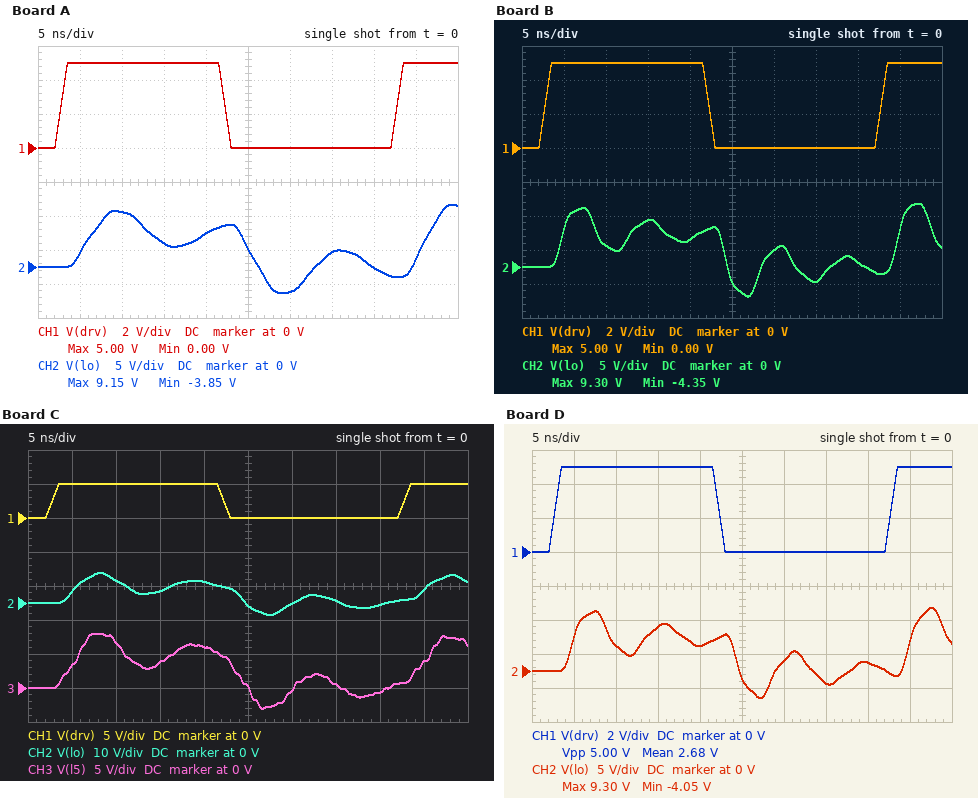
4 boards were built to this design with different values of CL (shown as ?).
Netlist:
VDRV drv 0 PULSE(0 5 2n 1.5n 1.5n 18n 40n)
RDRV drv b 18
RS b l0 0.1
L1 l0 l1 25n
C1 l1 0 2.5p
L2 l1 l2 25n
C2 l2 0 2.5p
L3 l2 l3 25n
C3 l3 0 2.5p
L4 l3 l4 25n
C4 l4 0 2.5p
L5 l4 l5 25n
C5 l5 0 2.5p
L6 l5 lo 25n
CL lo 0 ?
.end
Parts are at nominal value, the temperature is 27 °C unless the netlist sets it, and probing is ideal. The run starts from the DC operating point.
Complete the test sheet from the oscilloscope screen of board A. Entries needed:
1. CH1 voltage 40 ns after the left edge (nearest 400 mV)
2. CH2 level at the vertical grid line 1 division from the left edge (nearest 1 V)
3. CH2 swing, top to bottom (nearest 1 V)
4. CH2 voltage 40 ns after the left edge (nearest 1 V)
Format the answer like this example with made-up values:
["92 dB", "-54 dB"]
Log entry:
["0 V", "2 V", "13 V", "0 V"]
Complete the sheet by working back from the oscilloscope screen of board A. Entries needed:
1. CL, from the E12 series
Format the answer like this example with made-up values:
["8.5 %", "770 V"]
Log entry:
["27 pF"]
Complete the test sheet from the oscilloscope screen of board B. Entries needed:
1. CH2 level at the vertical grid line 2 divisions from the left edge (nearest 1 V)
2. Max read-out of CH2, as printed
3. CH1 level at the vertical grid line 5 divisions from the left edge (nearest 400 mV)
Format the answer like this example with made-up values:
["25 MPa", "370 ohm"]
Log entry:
["3 V", "9.30 V", "0 V"]
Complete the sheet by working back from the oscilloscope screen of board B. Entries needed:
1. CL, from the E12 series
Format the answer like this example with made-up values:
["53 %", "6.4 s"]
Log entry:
["6.8 pF"]
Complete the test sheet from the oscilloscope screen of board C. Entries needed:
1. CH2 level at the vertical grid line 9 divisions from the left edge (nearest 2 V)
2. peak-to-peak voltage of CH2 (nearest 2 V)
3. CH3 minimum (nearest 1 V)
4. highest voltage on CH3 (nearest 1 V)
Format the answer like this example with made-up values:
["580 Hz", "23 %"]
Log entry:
["4 V", "12 V", "-3 V", "8 V"]
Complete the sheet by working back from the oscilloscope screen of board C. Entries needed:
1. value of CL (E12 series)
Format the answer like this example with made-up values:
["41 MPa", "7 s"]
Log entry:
["15 pF"]
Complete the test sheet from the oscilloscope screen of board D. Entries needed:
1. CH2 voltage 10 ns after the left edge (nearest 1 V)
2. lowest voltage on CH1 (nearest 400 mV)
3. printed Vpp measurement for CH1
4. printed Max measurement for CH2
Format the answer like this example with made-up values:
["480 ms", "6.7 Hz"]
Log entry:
["4 V", "0 V", "5.00 V", "9.30 V"]
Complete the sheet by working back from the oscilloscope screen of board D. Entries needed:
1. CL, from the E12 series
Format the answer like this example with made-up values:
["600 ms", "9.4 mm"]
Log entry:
["8.2 pF"]
